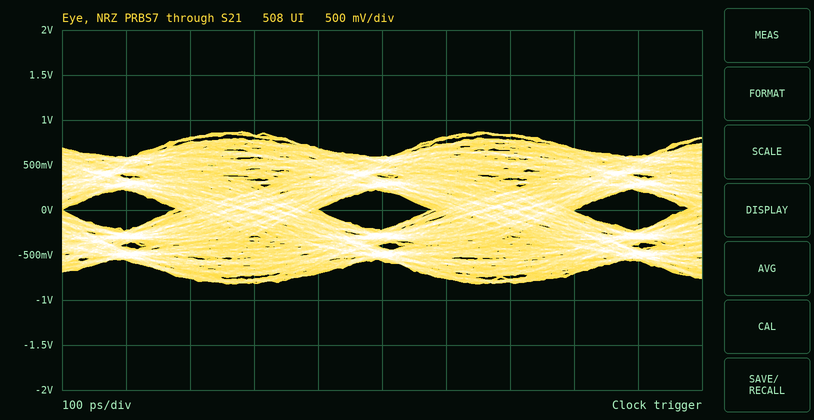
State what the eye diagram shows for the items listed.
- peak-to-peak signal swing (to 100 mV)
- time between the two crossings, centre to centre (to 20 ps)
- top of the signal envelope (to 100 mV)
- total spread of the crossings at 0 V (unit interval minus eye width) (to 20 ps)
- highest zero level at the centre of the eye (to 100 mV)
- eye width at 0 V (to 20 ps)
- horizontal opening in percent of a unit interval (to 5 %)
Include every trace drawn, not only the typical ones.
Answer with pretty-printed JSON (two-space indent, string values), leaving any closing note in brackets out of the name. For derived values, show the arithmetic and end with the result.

{
  "peak-to-peak signal swing": "1.7 V",
  "time between the two crossings, centre to centre": "400 ps",
  "top of the signal envelope": "900 mV",
  "total spread of the crossings at 0 V (unit interval minus eye width)": "220 ps",
  "highest zero level at the centre of the eye": "-200 mV",
  "eye width at 0 V": "180 ps",
  "horizontal opening in percent of a unit interval": "180 ps / 400 ps ≈ 45 %"
}
